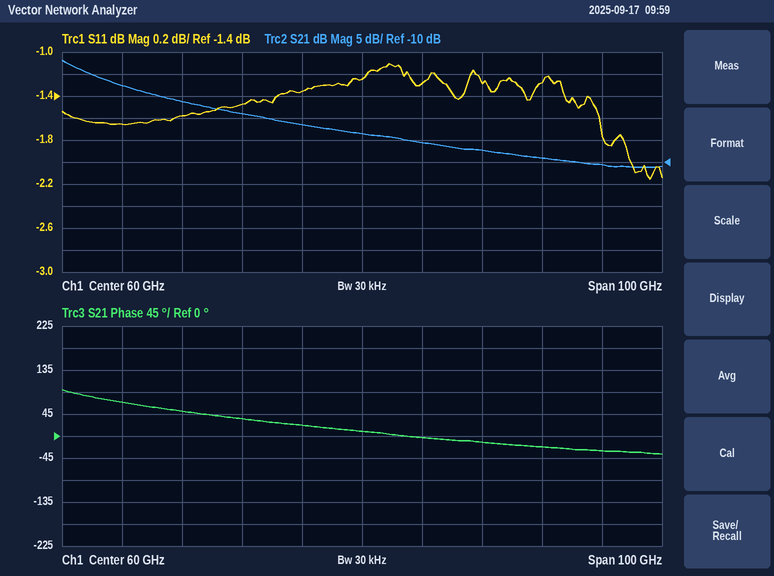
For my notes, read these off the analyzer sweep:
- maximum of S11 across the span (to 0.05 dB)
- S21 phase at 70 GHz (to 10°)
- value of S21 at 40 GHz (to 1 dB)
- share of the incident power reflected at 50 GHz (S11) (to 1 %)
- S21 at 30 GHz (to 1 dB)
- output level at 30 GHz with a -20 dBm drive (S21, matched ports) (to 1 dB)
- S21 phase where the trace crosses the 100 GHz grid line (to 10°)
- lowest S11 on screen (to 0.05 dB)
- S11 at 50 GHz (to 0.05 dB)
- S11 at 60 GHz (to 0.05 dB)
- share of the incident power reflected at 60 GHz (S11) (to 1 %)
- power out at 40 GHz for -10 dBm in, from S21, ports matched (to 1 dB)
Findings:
-1.10 dB
0°
1 dB
73 %
4 dB
-16 dBm
-30°
-2.15 dB
-1.35 dB
-1.25 dB
75 %
-9 dBm
